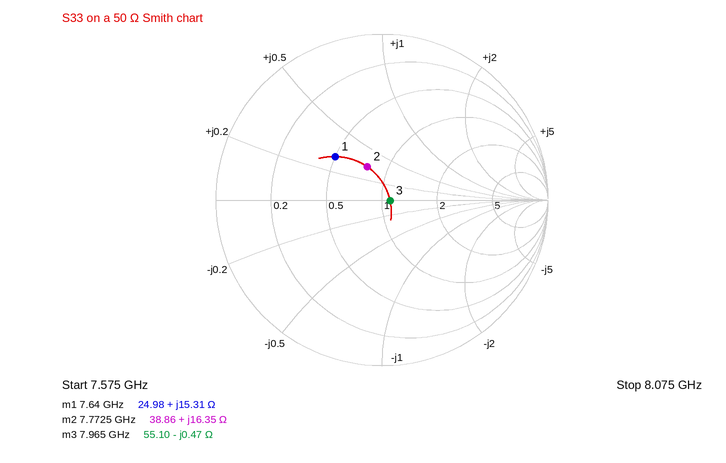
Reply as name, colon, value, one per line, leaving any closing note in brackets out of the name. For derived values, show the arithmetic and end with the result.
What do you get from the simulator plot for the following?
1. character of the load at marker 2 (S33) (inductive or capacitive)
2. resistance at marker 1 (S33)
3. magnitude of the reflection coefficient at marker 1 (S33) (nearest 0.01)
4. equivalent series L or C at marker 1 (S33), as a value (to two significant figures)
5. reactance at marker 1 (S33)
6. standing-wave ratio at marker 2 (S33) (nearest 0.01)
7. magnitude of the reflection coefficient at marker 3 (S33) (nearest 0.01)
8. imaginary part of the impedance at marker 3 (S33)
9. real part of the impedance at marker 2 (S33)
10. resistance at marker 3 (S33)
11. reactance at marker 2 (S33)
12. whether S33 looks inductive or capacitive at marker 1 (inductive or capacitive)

character of the load at marker 2 (S33): inductive
resistance at marker 1: 24.98 Ω
magnitude of the reflection coefficient at marker 1 (S33): 0.38
equivalent series L or C at marker 1 (S33), as a value: L = 15.31 Ω/(2π × 7.64 GHz) ≈ 319 pH, so 320 pH to two significant figures
reactance at marker 1: +15.31 Ω
standing-wave ratio at marker 2 (S33): 1.56
magnitude of the reflection coefficient at marker 3 (S33): 0.05
imaginary part of the impedance at marker 3: -0.47 Ω
real part of the impedance at marker 2: 38.86 Ω
resistance at marker 3: 55.10 Ω
reactance at marker 2: +16.35 Ω
whether S33 looks inductive or capacitive at marker 1: inductive
